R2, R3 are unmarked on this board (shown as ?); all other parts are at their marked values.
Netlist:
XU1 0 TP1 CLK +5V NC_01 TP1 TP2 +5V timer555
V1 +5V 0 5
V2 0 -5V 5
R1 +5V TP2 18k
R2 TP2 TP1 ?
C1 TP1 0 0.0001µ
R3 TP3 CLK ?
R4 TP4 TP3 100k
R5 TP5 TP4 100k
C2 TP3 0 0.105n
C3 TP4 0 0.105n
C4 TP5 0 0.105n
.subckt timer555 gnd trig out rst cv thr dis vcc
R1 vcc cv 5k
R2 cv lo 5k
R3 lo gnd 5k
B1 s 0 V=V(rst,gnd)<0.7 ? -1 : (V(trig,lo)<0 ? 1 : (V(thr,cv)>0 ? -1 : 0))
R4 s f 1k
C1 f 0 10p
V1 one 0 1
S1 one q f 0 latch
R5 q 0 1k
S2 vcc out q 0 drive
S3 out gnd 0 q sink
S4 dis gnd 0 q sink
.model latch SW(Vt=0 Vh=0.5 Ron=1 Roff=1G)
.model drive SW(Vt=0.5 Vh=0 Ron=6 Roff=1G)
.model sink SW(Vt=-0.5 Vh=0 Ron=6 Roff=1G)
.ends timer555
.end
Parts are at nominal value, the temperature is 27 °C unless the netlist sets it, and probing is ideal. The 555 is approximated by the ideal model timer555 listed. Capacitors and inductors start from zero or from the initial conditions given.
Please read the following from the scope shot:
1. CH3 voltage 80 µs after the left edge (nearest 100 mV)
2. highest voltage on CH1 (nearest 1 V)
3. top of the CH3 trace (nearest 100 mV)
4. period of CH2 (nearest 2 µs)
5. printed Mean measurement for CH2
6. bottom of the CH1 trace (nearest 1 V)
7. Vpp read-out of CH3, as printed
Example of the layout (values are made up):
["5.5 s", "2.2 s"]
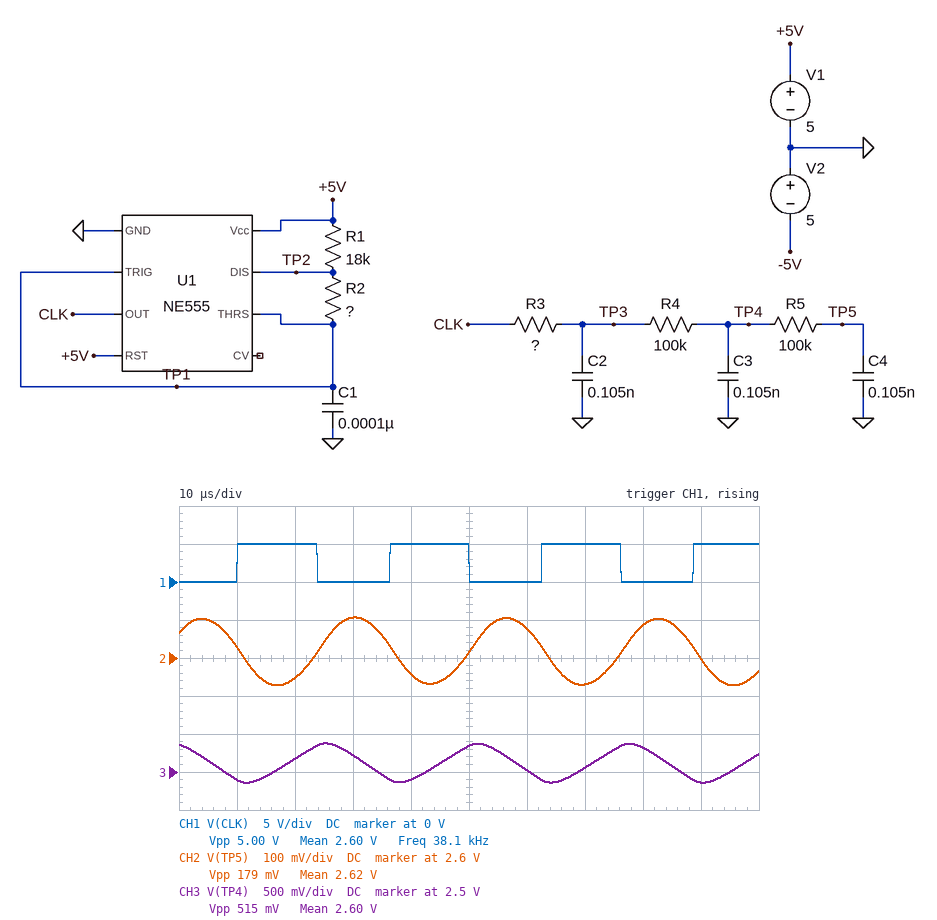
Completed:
["2.8 V", "5 V", "2.9 V", "26 µs", "2.62 V", "0 V", "515 mV"]
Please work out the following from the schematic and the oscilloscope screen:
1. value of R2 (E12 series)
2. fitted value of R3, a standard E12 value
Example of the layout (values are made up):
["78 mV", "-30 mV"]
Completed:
["180 kΩ", "120 kΩ"]
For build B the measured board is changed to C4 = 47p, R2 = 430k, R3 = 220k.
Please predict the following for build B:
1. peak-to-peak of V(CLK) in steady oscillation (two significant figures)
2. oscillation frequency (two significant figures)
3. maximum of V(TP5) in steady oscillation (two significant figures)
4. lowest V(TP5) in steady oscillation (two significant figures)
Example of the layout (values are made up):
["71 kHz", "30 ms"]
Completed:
["5.0 V", "16 kHz", "2.9 V", "2.2 V"]
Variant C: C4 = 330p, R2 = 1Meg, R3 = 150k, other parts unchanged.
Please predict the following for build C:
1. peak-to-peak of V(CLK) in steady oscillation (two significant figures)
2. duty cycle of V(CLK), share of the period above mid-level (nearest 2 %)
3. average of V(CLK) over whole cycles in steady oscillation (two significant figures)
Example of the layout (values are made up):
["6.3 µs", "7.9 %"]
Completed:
["5.0 V", "50 %", "2.5 V"]
